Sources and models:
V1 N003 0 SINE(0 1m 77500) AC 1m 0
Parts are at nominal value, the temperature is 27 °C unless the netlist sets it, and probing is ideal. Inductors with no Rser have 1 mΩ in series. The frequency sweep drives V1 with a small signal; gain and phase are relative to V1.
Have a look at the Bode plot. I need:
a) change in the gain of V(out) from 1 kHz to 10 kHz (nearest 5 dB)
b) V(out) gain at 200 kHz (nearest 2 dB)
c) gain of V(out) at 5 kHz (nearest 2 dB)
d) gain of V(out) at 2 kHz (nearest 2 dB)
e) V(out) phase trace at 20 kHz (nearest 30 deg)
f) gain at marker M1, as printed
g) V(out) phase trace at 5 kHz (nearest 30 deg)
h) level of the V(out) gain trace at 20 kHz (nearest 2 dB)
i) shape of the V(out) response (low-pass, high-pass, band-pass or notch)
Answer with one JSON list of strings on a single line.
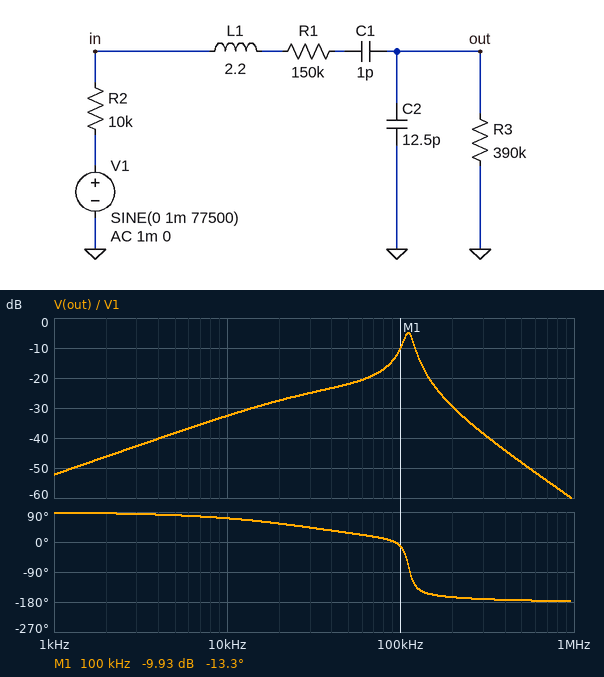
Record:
["20 dB", "-30 dB", "-38 dB", "-46 dB", "60 deg", "-9.93 dB", "90 deg", "-28 dB", "band-pass"]
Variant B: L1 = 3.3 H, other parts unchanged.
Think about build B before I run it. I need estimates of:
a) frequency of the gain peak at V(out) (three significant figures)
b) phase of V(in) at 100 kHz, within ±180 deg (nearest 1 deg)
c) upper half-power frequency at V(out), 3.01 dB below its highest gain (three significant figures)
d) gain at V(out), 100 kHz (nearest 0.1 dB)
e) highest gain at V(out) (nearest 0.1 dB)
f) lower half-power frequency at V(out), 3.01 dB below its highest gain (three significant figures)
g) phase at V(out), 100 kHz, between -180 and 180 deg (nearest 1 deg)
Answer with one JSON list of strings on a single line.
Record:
["90.5 kHz", "1 deg", "95.4 kHz", "-10.7 dB", "-3.8 dB", "85.4 kHz", "-134 deg"]
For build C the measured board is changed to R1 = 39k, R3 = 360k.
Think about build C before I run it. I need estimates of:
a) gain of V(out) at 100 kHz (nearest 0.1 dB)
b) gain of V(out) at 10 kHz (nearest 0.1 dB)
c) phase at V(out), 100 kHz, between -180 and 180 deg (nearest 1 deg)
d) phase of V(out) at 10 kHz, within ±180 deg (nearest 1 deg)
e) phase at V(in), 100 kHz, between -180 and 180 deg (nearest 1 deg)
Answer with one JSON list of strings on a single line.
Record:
["-8.9 dB", "-33.2 dB", "4 deg", "73 deg", "-2 deg"]
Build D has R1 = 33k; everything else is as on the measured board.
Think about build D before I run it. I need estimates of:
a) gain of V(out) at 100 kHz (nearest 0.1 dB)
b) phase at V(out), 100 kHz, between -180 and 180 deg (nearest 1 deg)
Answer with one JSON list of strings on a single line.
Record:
["-8.8 dB", "4 deg"]
